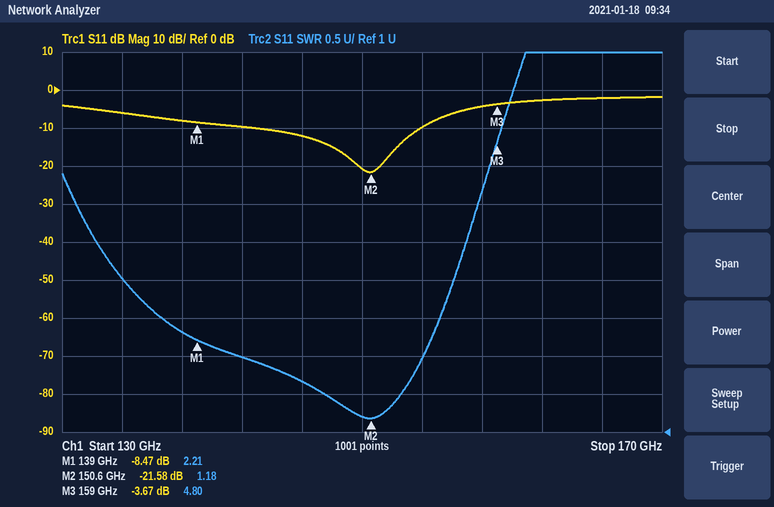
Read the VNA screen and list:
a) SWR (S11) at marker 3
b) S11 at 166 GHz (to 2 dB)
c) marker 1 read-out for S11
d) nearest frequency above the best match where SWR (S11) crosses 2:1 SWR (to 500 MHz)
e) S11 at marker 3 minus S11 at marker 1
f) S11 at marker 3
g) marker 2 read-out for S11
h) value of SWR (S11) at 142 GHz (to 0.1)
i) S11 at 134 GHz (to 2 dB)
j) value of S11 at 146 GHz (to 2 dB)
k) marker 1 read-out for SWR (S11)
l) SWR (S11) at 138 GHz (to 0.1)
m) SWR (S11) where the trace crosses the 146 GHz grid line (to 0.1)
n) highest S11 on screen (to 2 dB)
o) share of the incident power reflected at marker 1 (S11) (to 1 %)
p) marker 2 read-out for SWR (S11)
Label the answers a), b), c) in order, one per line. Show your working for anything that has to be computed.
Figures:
a) 4.80
b) -2 dB
c) -8.47 dB
d) 154.0 GHz
e) -3.67 − (-8.47) = 4.80 dB
f) -3.67 dB
g) -21.58 dB
h) 2.0
i) -6 dB
j) -12 dB
k) 2.21
l) 2.3
m) 1.7
n) -2 dB
o) 10^(-8.47/10) ≈ 14 %
p) 1.18
